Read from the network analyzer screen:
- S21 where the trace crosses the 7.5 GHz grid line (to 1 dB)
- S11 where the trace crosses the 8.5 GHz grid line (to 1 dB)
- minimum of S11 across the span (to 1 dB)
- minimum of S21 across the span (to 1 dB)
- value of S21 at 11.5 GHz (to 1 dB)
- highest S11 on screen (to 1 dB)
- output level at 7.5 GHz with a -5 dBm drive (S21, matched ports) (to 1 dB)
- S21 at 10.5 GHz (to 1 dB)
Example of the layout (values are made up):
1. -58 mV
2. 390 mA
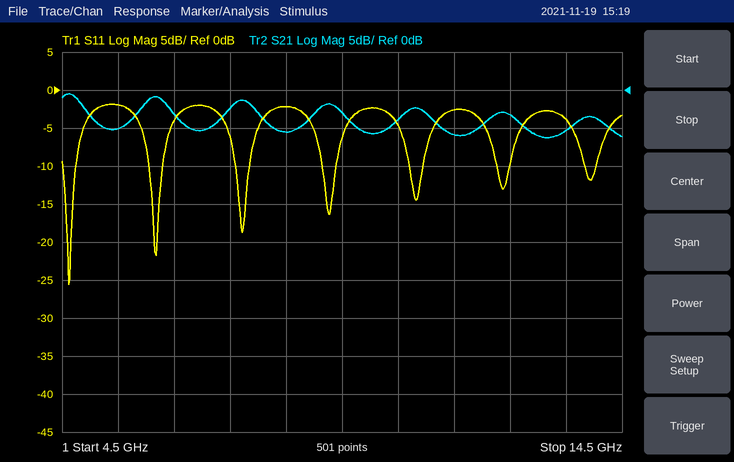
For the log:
1. -2 dB
2. -2 dB
3. -26 dB
4. -6 dB
5. -6 dB
6. -2 dB
7. -7 dBm
8. -4 dB
